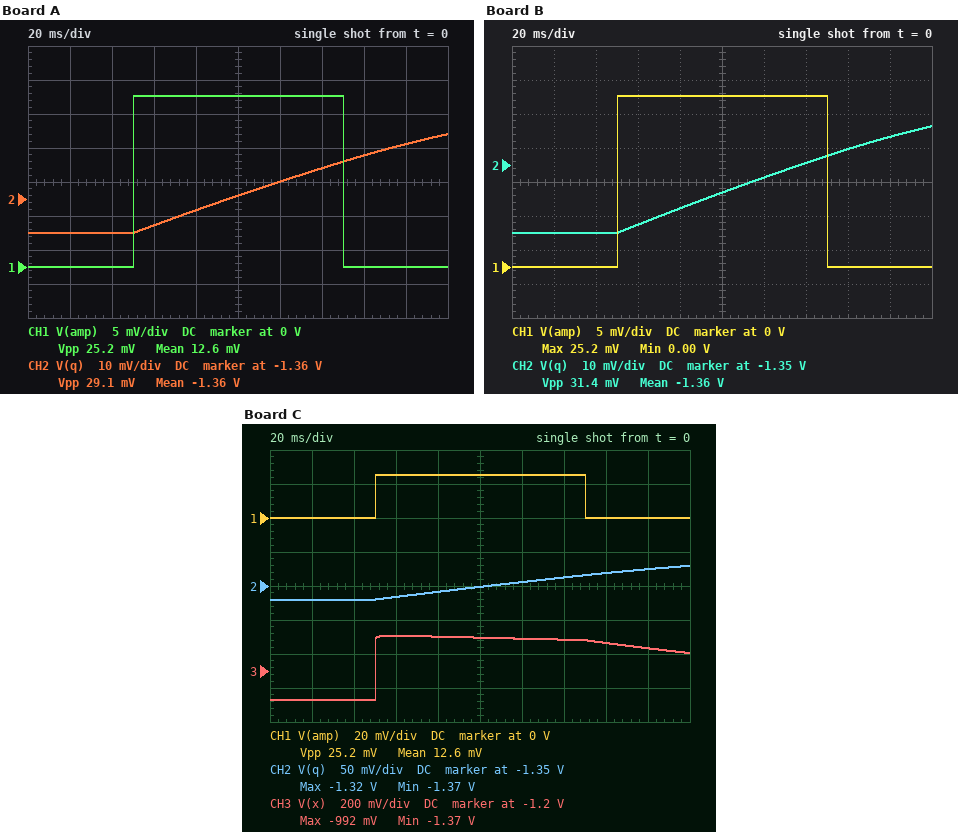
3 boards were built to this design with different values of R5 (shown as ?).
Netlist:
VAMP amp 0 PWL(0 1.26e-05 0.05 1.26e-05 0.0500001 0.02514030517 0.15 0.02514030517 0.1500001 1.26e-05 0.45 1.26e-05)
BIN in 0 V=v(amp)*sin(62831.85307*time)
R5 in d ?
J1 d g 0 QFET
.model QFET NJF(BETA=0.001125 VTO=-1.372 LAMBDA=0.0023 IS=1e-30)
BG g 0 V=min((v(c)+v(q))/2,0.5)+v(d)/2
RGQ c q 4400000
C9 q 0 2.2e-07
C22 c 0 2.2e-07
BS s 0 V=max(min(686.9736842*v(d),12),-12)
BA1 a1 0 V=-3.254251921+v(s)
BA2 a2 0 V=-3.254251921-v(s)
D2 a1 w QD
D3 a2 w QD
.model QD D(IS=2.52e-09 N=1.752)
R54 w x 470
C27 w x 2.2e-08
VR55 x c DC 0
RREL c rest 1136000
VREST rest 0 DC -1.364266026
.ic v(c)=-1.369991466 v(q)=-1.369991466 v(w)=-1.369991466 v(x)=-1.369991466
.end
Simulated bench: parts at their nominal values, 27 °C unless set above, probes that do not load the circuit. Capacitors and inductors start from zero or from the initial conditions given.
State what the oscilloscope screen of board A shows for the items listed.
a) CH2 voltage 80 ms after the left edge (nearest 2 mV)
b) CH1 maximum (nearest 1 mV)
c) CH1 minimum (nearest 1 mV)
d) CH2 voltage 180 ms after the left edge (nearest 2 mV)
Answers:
-1.364 V
25 mV
0 V
-1.344 V
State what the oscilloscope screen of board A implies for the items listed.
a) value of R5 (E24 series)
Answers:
24 kΩ
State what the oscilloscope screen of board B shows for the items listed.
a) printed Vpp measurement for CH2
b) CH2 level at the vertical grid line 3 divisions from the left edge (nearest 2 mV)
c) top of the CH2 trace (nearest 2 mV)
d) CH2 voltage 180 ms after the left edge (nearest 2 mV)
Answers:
31.4 mV
-1.368 V
-1.338 V
-1.342 V
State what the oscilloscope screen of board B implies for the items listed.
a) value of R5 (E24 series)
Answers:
22 kΩ
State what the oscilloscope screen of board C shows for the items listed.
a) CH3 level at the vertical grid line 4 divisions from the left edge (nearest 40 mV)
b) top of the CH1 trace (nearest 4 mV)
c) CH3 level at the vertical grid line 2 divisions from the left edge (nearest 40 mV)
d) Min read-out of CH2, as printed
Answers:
-1.00 V
24 mV
-1.36 V
-1.37 V
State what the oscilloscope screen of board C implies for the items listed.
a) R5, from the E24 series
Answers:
13 kΩ
